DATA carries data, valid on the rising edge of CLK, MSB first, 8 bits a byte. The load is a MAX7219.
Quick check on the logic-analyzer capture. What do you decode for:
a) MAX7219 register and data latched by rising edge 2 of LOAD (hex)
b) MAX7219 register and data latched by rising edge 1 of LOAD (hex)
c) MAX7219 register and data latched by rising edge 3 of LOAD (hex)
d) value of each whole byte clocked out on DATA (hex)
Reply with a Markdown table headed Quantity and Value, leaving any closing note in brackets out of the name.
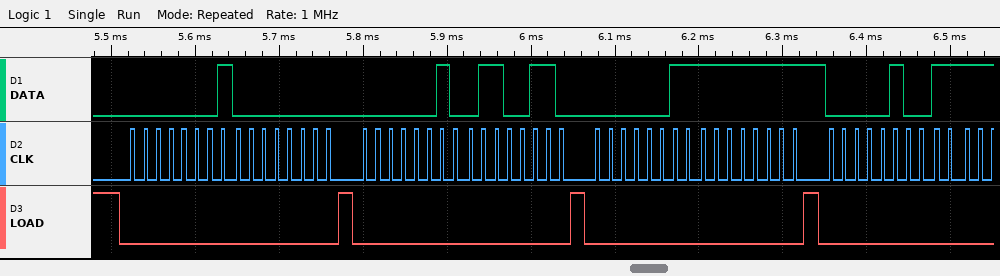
| Quantity | Value |
|---|---|
| MAX7219 register and data latched by rising edge 2 of LOAD | register 0x2, data 0x66 |
| MAX7219 register and data latched by rising edge 1 of LOAD | register 0x1, data 0x00 |
| MAX7219 register and data latched by rising edge 3 of LOAD | register 0x3, data 0xFF |
| value of each whole byte clocked out on DATA | 0x01 0x00 0x02 0x66 0x03 0xFF 0x04 |
